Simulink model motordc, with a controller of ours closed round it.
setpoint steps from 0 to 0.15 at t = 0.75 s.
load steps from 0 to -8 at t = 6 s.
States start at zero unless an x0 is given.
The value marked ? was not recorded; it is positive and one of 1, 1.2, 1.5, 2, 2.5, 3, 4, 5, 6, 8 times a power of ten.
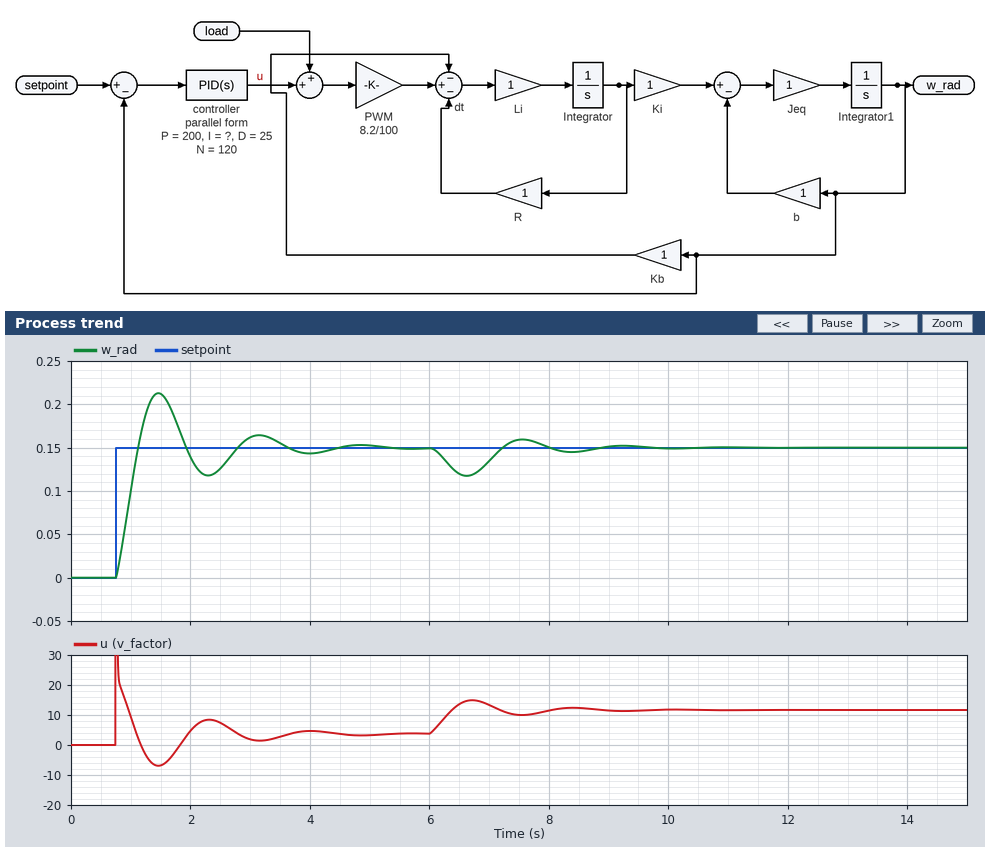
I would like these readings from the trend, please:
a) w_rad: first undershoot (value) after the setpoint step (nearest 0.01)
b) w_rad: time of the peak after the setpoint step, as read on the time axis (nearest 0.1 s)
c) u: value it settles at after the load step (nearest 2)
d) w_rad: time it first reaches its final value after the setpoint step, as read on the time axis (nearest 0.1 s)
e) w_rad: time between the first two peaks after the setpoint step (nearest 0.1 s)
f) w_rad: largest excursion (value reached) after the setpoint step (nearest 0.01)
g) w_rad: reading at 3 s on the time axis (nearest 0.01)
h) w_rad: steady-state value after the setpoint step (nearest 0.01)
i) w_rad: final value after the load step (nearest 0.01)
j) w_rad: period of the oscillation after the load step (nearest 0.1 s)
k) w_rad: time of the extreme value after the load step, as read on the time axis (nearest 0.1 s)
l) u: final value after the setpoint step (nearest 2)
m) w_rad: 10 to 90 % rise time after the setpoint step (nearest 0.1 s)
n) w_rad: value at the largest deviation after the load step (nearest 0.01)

0.12
1.5 s
12
1.1 s
1.7 s
0.21
0.16
0.15
0.15
1.8 s
6.6 s
4
0.3 s
0.12
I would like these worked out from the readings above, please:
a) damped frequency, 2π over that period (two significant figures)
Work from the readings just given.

3.7 rad/s
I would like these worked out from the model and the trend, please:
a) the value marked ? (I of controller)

400
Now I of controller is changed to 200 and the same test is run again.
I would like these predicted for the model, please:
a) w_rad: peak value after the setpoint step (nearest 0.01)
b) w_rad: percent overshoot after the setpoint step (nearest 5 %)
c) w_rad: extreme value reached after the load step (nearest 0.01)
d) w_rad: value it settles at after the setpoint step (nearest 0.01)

0.19
25 %
0.11
0.15
